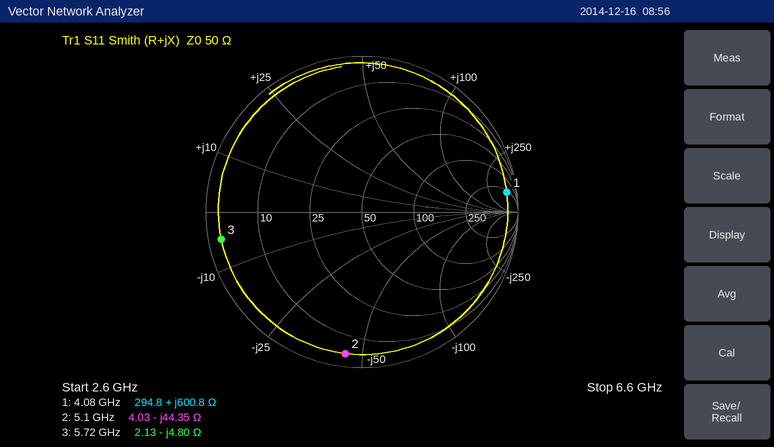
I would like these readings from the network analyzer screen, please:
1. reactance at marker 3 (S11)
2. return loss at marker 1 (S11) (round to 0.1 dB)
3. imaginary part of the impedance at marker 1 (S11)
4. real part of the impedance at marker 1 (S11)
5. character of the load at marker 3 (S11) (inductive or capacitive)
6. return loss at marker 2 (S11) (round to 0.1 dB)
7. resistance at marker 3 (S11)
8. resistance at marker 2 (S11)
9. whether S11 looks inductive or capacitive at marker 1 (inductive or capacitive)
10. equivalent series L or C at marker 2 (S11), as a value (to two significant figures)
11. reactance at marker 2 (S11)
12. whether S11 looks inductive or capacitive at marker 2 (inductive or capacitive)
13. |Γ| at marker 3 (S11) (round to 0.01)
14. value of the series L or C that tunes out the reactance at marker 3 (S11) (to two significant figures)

-4.80 Ω
0.6 dB
+600.8 Ω
294.8 Ω
capacitive
0.8 dB
2.13 Ω
4.03 Ω
inductive
700 fF
-44.35 Ω
capacitive
0.92
130 pH
